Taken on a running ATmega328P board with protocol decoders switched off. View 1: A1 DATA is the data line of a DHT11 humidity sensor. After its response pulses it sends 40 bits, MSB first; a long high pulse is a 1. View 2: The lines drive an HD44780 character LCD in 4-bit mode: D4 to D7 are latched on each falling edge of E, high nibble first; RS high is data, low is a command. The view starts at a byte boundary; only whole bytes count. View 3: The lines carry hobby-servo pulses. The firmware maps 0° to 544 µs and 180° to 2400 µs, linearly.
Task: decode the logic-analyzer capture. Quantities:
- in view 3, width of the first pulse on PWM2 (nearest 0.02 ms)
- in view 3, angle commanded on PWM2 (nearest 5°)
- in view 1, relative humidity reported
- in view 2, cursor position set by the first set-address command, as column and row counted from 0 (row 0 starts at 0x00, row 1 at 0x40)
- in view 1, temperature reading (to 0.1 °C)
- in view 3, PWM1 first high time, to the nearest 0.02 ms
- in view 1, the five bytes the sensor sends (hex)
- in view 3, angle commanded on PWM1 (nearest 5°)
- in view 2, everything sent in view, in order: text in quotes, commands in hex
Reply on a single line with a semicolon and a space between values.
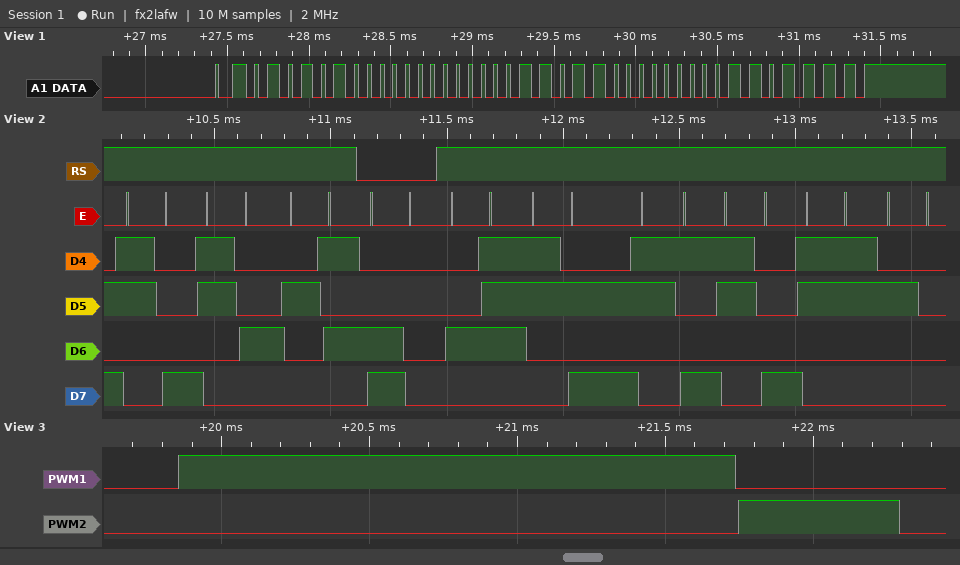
0.54 ms; 0°; 84 %; column 0, row 1; 27.0 °C; 1.88 ms; 54 00 1B 00 6F; 130°; "84%" 0xC0 "G:983 "
